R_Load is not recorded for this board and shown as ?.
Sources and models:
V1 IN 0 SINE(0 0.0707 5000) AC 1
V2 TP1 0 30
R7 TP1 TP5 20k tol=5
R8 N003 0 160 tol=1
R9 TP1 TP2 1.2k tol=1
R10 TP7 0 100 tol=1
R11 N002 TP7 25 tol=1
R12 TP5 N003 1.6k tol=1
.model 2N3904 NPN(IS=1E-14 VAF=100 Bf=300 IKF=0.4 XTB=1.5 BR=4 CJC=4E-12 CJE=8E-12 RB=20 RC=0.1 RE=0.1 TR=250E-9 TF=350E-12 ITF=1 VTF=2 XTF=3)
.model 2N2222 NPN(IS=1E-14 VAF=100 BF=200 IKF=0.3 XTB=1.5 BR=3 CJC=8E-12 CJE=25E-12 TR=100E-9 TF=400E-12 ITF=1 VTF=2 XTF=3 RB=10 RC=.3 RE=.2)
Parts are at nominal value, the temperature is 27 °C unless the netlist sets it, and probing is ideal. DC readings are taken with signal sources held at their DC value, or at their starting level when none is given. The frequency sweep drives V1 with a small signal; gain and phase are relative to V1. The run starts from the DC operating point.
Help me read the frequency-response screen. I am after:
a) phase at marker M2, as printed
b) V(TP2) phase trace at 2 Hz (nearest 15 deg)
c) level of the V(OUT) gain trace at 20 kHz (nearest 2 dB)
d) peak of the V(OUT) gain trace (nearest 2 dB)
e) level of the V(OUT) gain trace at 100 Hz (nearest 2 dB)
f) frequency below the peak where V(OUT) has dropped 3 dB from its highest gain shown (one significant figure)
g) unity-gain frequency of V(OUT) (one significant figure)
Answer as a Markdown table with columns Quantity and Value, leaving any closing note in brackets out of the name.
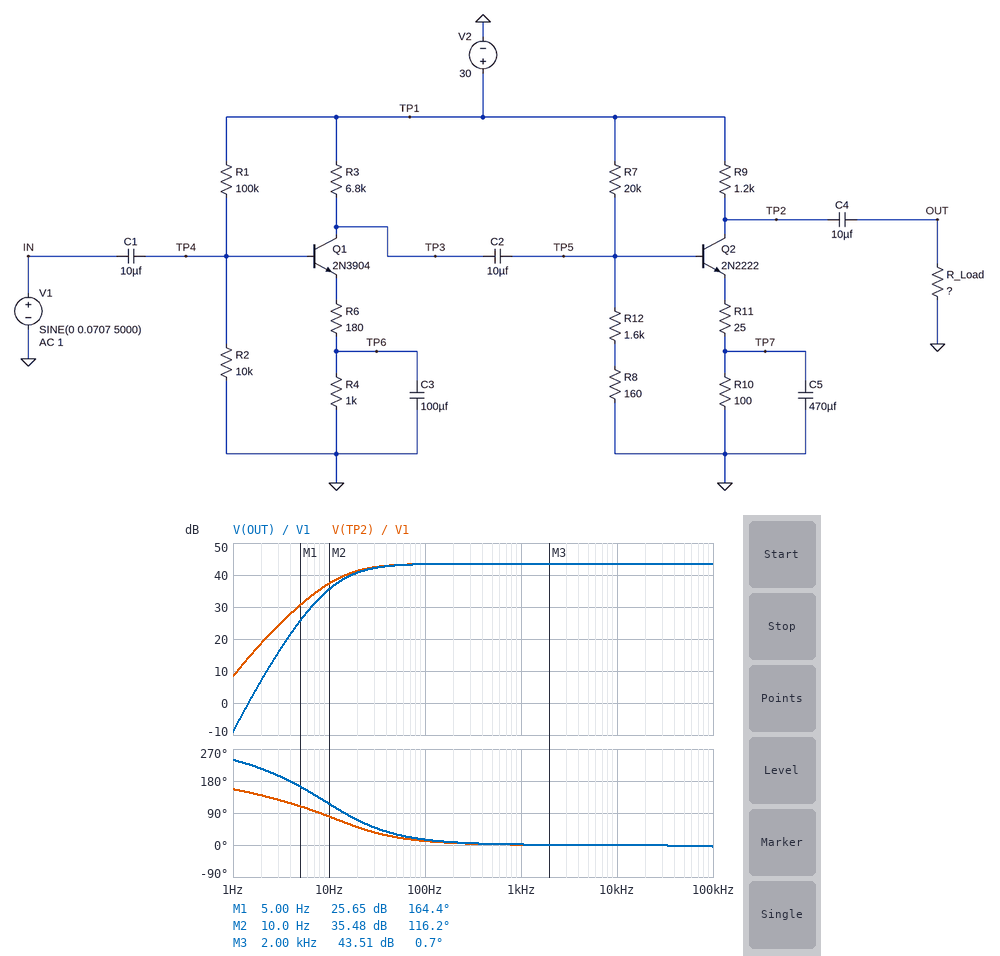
| Quantity | Value |
|---|---|
| phase at marker M2, as printed | 116.2 deg |
| V(TP2) phase trace at 2 Hz | 135 deg |
| level of the V(OUT) gain trace at 20 kHz | 44 dB |
| peak of the V(OUT) gain trace | 44 dB |
| level of the V(OUT) gain trace at 100 Hz | 44 dB |
| frequency below the peak where V(OUT) has dropped 3 dB from its highest gain shown | 20 Hz |
| unity-gain frequency of V(OUT) | 1 Hz |
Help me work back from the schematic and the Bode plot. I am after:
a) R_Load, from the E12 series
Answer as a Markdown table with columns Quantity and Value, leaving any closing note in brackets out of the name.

| Quantity | Value |
|---|---|
| R_Load, from the E12 series | 2.2 kΩ |
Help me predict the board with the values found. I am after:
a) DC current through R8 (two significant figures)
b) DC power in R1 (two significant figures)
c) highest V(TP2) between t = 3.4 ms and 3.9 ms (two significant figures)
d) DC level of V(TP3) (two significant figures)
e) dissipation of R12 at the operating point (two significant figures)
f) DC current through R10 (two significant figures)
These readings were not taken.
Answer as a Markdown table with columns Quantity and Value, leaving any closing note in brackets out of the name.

| Quantity | Value |
|---|---|
| DC current through R8 | 1.3 mA |
| DC power in R1 | 7.5 mW |
| highest V(TP2) between t = 3.4 ms and 3.9 ms | 24 V |
| DC level of V(TP3) | 18 V |
| dissipation of R12 at the operating point | 2.8 mW |
| DC current through R10 | 13 mA |
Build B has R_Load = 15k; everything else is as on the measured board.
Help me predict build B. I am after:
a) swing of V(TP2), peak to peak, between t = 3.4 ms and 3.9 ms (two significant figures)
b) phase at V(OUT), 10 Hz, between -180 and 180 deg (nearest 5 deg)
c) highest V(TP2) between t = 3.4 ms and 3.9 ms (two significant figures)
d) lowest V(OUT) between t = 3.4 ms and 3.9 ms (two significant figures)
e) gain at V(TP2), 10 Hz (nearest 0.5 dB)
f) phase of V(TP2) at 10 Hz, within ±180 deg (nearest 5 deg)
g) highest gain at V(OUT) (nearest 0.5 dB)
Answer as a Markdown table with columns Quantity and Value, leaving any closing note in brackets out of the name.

| Quantity | Value |
|---|---|
| swing of V(TP2), peak to peak, between t = 3.4 ms and 3.9 ms | 26 V |
| phase at V(OUT), 10 Hz, between -180 and 180 deg | 95 deg |
| highest V(TP2) between t = 3.4 ms and 3.9 ms | 28 V |
| lowest V(OUT) between t = 3.4 ms and 3.9 ms | -13 V |
| gain at V(TP2), 10 Hz | 39.5 dB |
| phase of V(TP2) at 10 Hz, within ±180 deg | 90 deg |
| highest gain at V(OUT) | 46.5 dB |
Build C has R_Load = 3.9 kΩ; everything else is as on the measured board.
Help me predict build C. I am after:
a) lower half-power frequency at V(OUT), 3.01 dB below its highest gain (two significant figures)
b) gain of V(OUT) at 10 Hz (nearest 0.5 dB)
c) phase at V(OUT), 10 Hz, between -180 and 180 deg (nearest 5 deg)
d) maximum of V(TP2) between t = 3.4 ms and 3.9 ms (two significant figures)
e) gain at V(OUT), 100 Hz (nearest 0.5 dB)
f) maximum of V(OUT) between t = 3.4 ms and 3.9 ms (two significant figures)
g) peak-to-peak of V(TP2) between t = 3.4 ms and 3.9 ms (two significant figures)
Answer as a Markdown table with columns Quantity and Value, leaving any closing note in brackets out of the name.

| Quantity | Value |
|---|---|
| lower half-power frequency at V(OUT), 3.01 dB below its highest gain | 18 Hz |
| gain of V(OUT) at 10 Hz | 37.5 dB |
| phase at V(OUT), 10 Hz, between -180 and 180 deg | 110 deg |
| maximum of V(TP2) between t = 3.4 ms and 3.9 ms | 26 V |
| gain at V(OUT), 100 Hz | 45.0 dB |
| maximum of V(OUT) between t = 3.4 ms and 3.9 ms | 11 V |
| peak-to-peak of V(TP2) between t = 3.4 ms and 3.9 ms | 23 V |
